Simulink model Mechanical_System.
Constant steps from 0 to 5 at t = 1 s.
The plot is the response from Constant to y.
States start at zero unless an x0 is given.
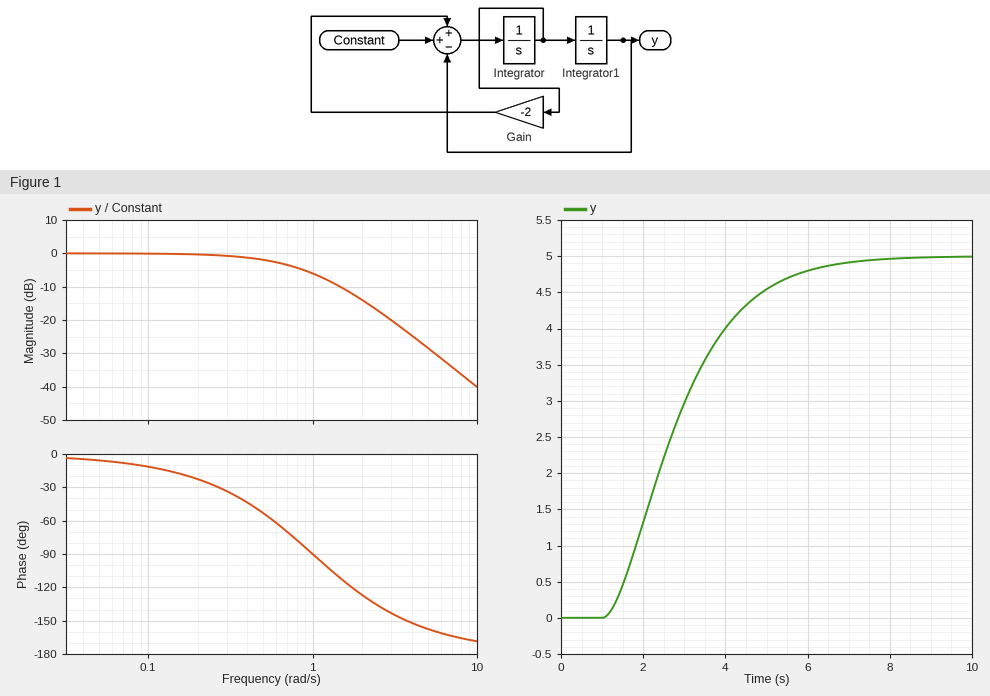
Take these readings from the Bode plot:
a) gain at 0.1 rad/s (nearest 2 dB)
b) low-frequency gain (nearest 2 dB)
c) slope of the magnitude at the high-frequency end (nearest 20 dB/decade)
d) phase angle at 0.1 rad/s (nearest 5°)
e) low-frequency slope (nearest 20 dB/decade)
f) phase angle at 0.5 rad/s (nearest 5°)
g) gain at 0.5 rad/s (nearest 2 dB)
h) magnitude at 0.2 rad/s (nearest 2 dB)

0 dB
0 dB
-40 dB/decade
-10°
0 dB/decade
-55°
-2 dB
0 dB
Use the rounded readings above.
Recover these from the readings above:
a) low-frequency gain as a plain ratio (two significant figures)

1.0
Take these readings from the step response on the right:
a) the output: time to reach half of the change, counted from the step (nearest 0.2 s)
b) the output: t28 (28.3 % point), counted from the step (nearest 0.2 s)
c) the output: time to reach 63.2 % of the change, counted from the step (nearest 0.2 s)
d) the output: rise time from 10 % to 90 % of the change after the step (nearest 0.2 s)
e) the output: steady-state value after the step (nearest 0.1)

1.6 s
1.0 s
2.2 s
3.4 s
5.0
